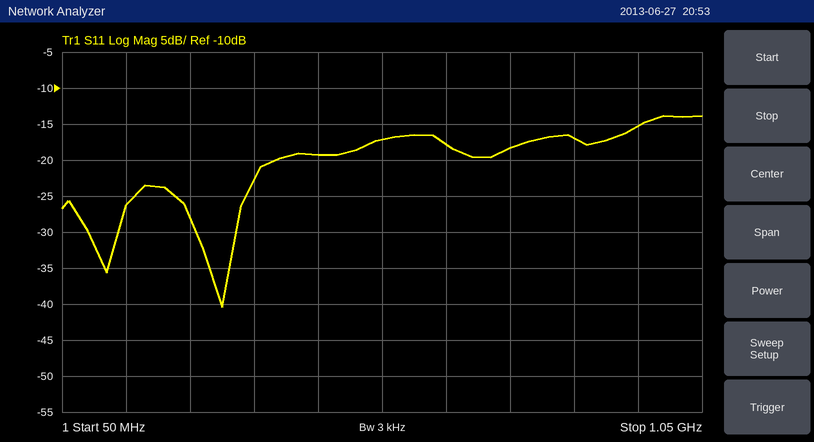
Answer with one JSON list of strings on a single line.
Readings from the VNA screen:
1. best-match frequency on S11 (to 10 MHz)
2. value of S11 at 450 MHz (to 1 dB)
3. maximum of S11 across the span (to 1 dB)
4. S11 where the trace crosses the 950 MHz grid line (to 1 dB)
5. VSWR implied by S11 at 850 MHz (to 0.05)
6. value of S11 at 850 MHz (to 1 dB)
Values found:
["300 MHz", "-19 dB", "-14 dB", "-15 dB", "1.35", "-17 dB"]
